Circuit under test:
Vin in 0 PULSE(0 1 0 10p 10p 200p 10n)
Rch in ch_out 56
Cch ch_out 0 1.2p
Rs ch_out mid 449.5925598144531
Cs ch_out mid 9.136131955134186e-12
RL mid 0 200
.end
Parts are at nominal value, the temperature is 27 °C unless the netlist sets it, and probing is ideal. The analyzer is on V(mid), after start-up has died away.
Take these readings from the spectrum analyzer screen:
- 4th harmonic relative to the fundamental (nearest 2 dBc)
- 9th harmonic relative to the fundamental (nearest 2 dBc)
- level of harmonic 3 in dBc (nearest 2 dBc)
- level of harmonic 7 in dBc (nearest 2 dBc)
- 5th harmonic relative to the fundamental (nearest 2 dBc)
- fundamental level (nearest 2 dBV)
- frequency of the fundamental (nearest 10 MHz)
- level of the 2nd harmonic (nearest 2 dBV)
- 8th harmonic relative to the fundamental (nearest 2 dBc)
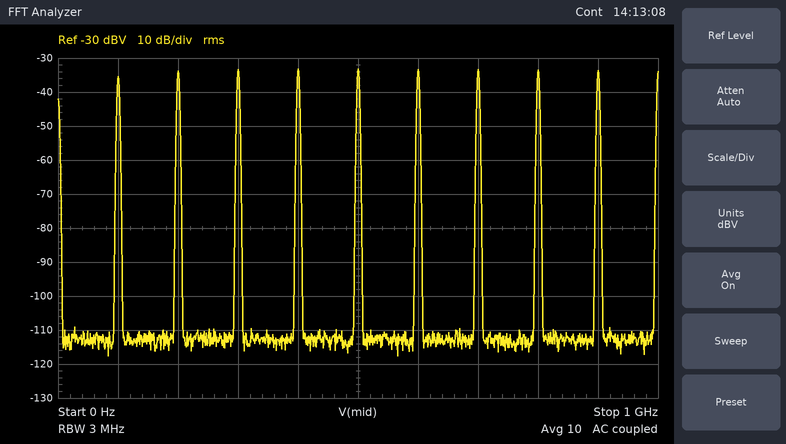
2 dBc
2 dBc
2 dBc
2 dBc
2 dBc
-36 dBV
100 MHz
-34 dBV
2 dBc
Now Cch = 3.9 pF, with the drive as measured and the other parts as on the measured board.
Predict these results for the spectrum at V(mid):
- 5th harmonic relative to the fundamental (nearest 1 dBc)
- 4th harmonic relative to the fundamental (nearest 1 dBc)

1 dBc
2 dBc
